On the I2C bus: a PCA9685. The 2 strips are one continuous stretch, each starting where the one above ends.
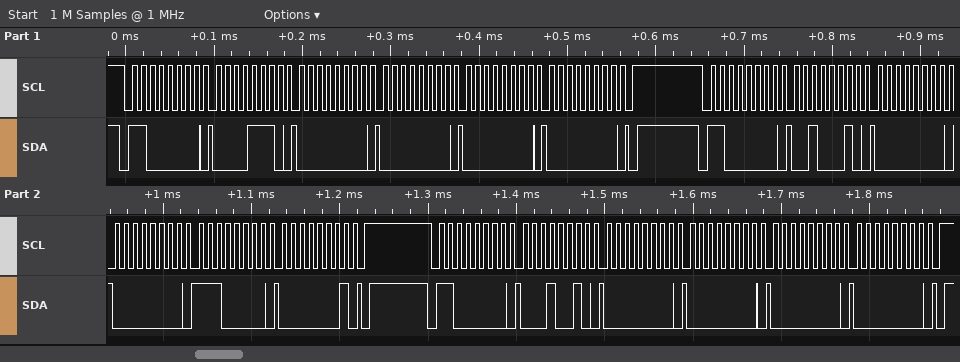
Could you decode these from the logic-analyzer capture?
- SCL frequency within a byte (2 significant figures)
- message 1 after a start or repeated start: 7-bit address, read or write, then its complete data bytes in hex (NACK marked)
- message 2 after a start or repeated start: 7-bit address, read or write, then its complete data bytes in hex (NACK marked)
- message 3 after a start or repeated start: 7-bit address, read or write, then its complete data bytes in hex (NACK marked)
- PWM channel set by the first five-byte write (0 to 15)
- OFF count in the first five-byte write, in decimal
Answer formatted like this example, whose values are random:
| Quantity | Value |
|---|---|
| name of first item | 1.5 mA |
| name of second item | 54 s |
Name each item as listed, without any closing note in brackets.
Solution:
| Quantity | Value |
|---|---|
| SCL frequency within a byte | 100 kHz |
| message 1 after a start or repeated start: 7-bit address, read or write, then its complete data bytes in hex | 0x60 write: 0E 00 00 00 00 |
| message 2 after a start or repeated start: 7-bit address, read or write, then its complete data bytes in hex | 0x60 write: 22 00 00 E0 01 |
| message 3 after a start or repeated start: 7-bit address, read or write, then its complete data bytes in hex | 0x60 write: 12 00 00 00 00 |
| PWM channel set by the first five-byte write | 2 |
| OFF count in the first five-byte write, in decimal | 0 |
